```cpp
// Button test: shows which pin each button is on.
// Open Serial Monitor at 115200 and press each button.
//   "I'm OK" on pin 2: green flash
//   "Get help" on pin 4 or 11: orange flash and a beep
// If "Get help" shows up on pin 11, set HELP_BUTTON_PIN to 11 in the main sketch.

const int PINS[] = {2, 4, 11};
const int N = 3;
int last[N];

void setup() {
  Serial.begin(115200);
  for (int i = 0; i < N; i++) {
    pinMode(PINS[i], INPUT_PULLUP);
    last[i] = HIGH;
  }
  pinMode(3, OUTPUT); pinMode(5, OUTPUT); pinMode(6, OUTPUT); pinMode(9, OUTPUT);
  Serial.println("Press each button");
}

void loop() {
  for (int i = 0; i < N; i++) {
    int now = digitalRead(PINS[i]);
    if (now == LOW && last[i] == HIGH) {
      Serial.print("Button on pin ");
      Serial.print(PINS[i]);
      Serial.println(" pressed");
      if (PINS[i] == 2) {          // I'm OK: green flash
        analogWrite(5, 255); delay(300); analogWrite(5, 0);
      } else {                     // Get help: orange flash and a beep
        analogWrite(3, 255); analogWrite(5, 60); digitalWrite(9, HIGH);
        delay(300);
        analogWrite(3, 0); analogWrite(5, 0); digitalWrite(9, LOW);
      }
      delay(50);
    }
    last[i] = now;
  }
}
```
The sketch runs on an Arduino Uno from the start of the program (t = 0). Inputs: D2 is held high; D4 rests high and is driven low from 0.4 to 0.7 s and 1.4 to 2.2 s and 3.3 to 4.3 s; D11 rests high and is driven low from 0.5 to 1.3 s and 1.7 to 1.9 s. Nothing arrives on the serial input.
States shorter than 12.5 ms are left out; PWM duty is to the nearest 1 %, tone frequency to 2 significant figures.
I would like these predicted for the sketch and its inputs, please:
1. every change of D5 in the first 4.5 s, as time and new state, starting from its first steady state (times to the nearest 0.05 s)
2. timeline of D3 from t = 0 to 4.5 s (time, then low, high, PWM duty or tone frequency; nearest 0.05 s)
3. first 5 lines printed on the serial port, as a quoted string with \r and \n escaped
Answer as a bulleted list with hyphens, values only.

- 0 s low; 0.4 s PWM 24 %; 0.7 s low; 0.75 s PWM 24 %; 1.05 s low; 1.4 s PWM 24 %; 1.7 s low; 1.75 s PWM 24 %; 2.05 s low; 3.3 s PWM 24 %; 3.6 s low
- 0 s low; 0.4 s high; 0.7 s low; 0.75 s high; 1.05 s low; 1.4 s high; 1.7 s low; 1.75 s high; 2.05 s low; 3.3 s high; 3.6 s low
- "Press each button\r\nButton on pin 4 pressed\r\nButton on pin 11 pressed\r\nButton on pin 4 pressed\r\nButton on pin 11 pressed\r\n"
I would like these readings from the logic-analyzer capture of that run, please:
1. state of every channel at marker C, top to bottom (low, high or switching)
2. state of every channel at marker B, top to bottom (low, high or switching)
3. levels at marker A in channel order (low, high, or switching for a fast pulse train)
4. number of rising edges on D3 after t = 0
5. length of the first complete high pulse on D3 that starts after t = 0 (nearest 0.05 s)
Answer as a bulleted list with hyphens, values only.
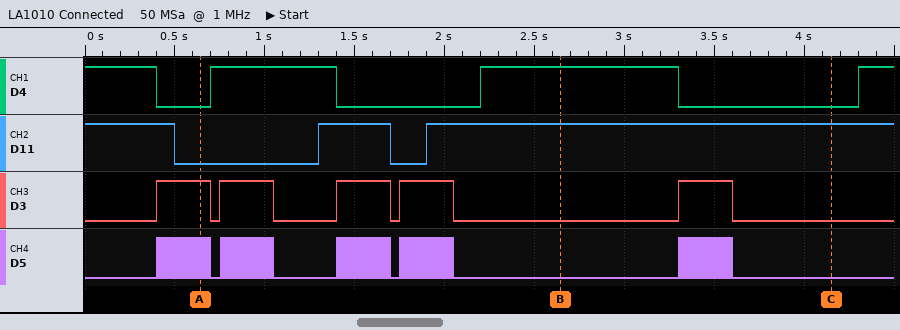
- D4 low, D11 high, D3 low, D5 low
- D4 high, D11 high, D3 low, D5 low
- D4 low, D11 low, D3 high, D5 switching
- 5
- 0.30 s
